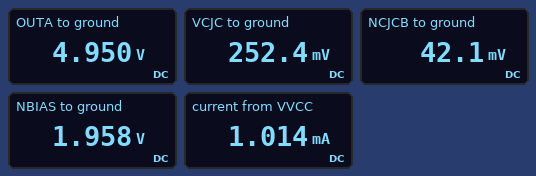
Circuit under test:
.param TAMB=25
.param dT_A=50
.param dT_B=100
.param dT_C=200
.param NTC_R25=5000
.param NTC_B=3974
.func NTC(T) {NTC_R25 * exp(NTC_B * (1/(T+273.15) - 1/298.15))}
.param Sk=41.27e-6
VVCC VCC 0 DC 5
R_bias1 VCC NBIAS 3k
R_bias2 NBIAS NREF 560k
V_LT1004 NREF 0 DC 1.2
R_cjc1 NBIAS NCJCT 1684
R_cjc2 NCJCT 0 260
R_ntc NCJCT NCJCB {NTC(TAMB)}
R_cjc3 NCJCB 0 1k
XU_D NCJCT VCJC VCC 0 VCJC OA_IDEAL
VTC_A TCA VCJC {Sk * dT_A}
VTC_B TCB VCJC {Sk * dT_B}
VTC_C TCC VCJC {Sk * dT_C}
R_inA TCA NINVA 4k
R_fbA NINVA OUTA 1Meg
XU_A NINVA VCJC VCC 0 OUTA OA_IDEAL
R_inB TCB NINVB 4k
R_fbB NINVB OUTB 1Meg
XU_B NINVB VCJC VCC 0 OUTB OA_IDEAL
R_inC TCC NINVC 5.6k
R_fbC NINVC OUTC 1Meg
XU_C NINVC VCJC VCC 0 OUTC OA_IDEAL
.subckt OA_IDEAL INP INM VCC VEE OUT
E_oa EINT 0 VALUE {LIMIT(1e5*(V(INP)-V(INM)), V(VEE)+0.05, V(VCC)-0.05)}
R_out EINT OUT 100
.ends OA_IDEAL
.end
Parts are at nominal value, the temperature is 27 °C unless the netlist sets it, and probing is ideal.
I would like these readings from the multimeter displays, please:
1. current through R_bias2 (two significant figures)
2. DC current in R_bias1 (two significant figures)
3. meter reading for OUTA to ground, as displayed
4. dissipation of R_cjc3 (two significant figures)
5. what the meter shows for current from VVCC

1.4 µA
1.0 mA
4.950 V
1.8 µW
1.014 mA
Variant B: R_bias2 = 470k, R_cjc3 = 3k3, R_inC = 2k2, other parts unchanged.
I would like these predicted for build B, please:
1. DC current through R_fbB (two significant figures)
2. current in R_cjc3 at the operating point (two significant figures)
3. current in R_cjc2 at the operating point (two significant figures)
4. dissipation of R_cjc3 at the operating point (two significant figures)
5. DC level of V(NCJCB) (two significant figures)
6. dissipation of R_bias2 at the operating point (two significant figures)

4.7 µA
31 µA
980 µA
3.1 µW
100 mV
1.2 µW
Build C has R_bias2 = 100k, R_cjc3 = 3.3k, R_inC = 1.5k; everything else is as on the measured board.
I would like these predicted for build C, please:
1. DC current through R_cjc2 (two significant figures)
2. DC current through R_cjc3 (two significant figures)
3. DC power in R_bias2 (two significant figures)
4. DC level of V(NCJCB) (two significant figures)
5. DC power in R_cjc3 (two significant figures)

980 µA
31 µA
5.7 µW
100 mV
3.1 µW
